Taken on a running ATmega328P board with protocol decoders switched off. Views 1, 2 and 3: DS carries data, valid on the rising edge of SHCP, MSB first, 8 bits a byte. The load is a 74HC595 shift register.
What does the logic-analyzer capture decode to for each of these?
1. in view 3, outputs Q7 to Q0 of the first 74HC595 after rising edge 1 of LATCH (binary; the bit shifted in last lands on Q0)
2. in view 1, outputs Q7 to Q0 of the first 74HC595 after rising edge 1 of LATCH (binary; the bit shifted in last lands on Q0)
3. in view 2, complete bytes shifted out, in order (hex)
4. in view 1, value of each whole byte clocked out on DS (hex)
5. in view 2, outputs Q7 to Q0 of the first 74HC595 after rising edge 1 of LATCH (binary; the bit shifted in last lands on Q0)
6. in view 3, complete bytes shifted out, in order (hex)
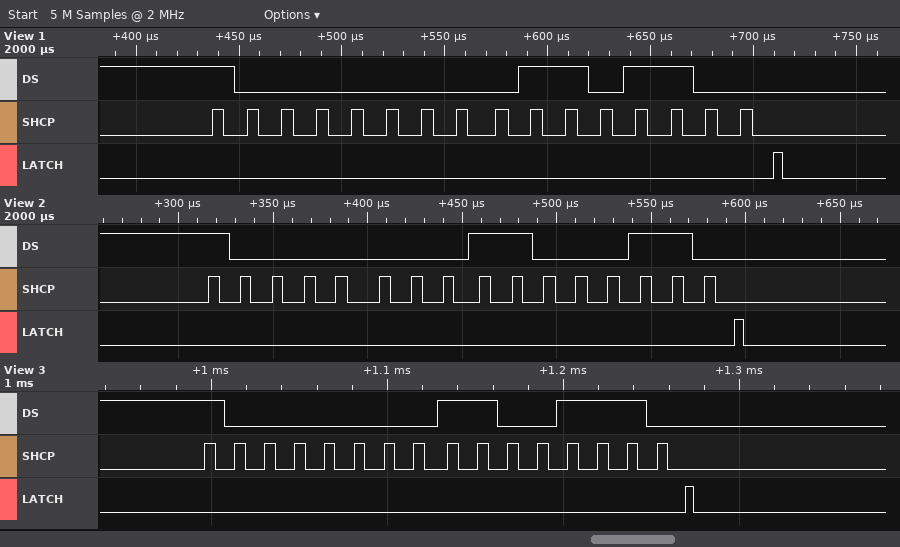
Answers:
11001110
01101100
80 C6
80 6C
11000110
0x80 0xCE
